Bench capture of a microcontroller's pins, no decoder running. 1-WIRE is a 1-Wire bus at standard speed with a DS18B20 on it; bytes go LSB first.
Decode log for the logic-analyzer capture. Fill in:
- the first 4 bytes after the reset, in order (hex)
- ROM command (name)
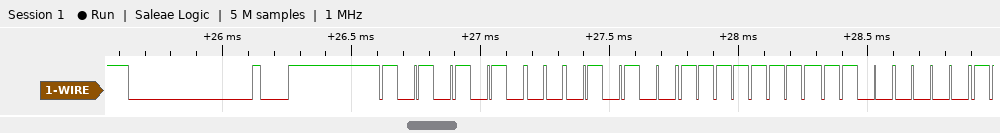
55 28 FF 03
Match ROM
